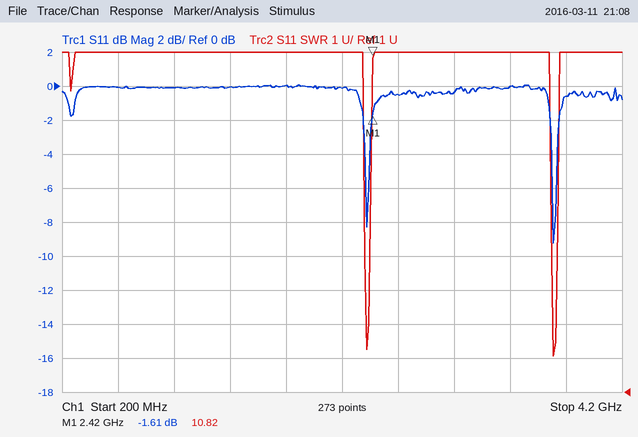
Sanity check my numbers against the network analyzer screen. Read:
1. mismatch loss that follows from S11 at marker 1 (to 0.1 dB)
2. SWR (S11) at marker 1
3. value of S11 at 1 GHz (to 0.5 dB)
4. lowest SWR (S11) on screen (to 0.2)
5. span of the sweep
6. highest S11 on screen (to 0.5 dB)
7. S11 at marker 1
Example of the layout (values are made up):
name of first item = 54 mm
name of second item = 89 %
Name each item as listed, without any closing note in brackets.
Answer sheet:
mismatch loss that follows from S11 at marker 1 = 5.1 dB
SWR (S11) at marker 1 = 10.82
value of S11 at 1 GHz = 0.0 dB
lowest SWR (S11) on screen = 2.0
span of the sweep = 4 GHz
highest S11 on screen = 0.0 dB
S11 at marker 1 = -1.61 dB
